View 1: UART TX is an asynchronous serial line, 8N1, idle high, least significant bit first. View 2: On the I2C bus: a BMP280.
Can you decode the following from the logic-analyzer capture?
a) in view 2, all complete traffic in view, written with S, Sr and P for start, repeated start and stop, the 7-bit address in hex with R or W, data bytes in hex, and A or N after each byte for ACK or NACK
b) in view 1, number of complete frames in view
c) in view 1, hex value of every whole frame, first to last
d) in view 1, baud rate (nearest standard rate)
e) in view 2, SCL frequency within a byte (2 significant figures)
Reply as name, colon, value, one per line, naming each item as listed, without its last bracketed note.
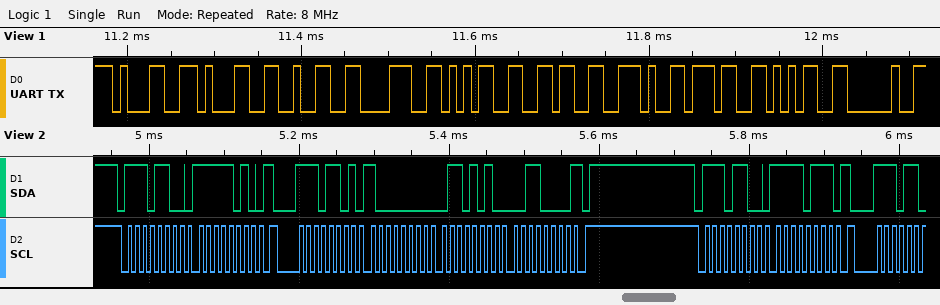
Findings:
in view 2, all complete traffic in view, written with S, Sr and P for start, repeated start and stop, the 7-bit address in hex with R or W, data bytes in hex, and A or N after each byte for ACK or NACK: S 76W A FA A Sr 76R A 80 A 6A A 30 N P S 76W A F7 A
in view 1, number of complete frames in view: 10
in view 1, hex value of every whole frame, first to last: 31 31 32 38 35 36 2E 37 35 20
in view 1, baud rate: 115200 baud
in view 2, SCL frequency within a byte: 100 kHz
